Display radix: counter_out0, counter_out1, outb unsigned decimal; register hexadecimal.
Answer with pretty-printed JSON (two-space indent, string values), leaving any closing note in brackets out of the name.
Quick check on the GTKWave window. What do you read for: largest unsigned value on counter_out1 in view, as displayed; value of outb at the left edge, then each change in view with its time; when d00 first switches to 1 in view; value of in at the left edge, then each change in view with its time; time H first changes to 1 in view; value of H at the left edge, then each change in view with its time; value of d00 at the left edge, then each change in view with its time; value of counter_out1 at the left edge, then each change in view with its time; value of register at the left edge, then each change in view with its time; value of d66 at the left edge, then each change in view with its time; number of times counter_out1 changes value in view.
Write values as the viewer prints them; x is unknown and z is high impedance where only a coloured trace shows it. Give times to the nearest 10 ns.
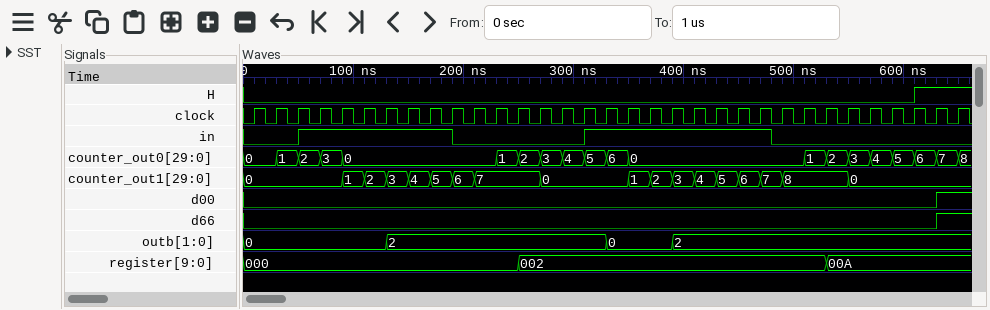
{
  "largest unsigned value on counter_out1 in view, as displayed": "8",
  "value of outb at the left edge, then each change in view with its time": "0, 2 at 130 ns, 0 at 330 ns, 2 at 390 ns",
  "when d00 first switches to 1 in view": "630 ns",
  "value of in at the left edge, then each change in view with its time": "0, 1 at 50 ns, 0 at 190 ns, 1 at 310 ns, 0 at 480 ns",
  "time H first changes to 1 in view": "610 ns",
  "value of H at the left edge, then each change in view with its time": "0, 1 at 610 ns",
  "value of d00 at the left edge, then each change in view with its time": "0, 1 at 630 ns",
  "value of counter_out1 at the left edge, then each change in view with its time": "0, 1 at 90 ns, 2 at 110 ns, 3 at 130 ns, 4 at 150 ns, 5 at 170 ns, 6 at 190 ns, 7 at 210 ns, 0 at 270 ns, 1 at 350 ns, 2 at 370 ns, 3 at 390 ns, 4 at 410 ns, 5 at 430 ns, 6 at 450 ns, 7 at 470 ns, 8 at 490 ns, 0 at 550 ns",
  "value of register at the left edge, then each change in view with its time": "000, 002 at 250 ns, 00A at 530 ns",
  "value of d66 at the left edge, then each change in view with its time": "0, 1 at 630 ns",
  "number of times counter_out1 changes value in view": "17"
}
